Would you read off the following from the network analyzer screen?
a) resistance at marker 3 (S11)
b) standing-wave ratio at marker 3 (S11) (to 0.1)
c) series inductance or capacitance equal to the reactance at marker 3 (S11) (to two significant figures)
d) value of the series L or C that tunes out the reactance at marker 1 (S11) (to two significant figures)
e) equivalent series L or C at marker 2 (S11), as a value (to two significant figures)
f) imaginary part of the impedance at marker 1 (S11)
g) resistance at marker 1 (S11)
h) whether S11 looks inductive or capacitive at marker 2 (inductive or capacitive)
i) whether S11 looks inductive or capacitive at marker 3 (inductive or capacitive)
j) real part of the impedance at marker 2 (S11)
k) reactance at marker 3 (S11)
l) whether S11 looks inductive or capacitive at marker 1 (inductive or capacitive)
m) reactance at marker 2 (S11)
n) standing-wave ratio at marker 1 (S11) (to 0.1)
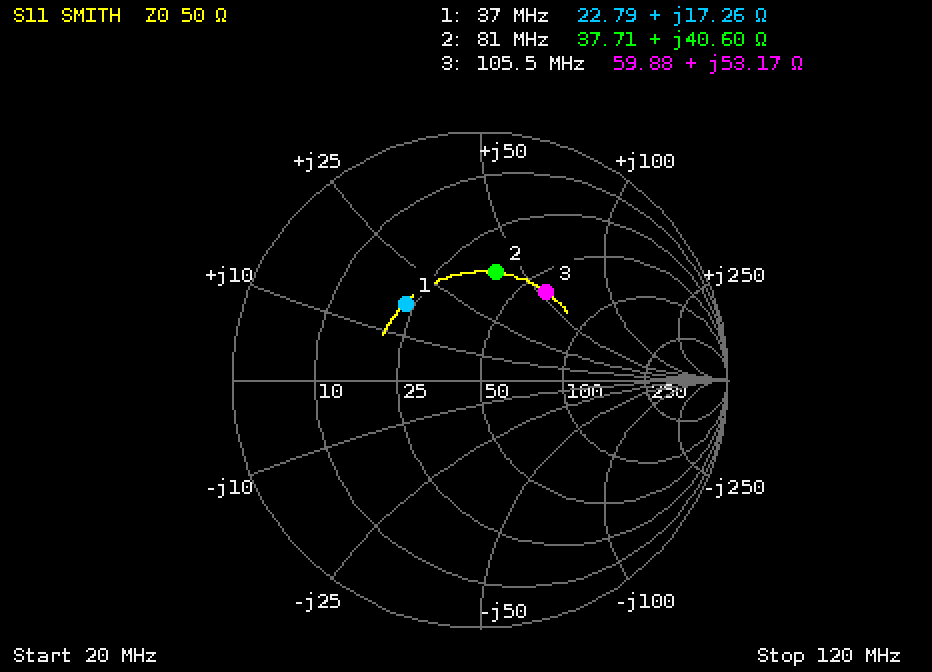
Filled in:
59.88 Ω
2.6
80 nH
250 pF
80 nH
+17.26 Ω
22.79 Ω
inductive
inductive
37.71 Ω
+53.17 Ω
inductive
+40.60 Ω
2.5
